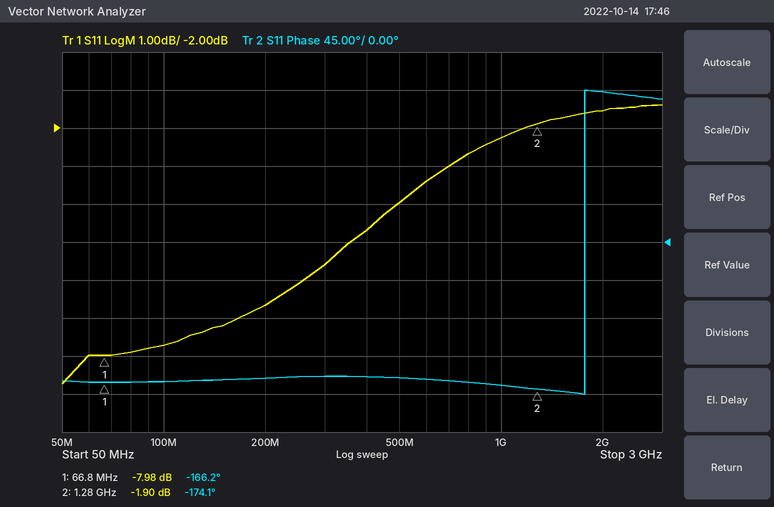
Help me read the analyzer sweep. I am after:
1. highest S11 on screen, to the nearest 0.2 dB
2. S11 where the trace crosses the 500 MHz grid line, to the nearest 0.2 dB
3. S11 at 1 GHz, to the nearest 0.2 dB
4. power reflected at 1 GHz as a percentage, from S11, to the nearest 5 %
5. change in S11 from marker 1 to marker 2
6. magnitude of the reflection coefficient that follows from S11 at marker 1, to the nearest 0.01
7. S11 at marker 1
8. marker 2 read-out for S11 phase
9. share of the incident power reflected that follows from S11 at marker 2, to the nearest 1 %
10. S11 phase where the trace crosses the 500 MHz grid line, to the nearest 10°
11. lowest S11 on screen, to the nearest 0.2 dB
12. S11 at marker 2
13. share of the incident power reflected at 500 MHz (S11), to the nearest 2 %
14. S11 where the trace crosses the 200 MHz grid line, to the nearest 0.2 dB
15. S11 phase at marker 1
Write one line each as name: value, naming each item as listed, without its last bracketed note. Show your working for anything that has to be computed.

highest S11 on screen, to the nearest 0.2 dB: -1.4 dB
S11 where the trace crosses the 500 MHz grid line, to the nearest 0.2 dB: -4.0 dB
S11 at 1 GHz, to the nearest 0.2 dB: -2.2 dB
power reflected at 1 GHz as a percentage, from S11, to the nearest 5 %: 10^(-2.2/10) ≈ 60 %
change in S11 from marker 1 to marker 2: -1.9 − (-7.98) = 6.08 dB
magnitude of the reflection coefficient that follows from S11 at marker 1, to the nearest 0.01: 10^(-7.98/20) ≈ 0.40
S11 at marker 1: -7.98 dB
marker 2 read-out for S11 phase: -174.1°
share of the incident power reflected that follows from S11 at marker 2, to the nearest 1 %: 10^(-1.9/10) ≈ 65 %
S11 phase where the trace crosses the 500 MHz grid line, to the nearest 10°: -160°
lowest S11 on screen, to the nearest 0.2 dB: -8.8 dB
S11 at marker 2: -1.90 dB
share of the incident power reflected at 500 MHz (S11), to the nearest 2 %: 10^(-4/10) ≈ 40 %
S11 where the trace crosses the 200 MHz grid line, to the nearest 0.2 dB: -6.6 dB
S11 phase at marker 1: -166.2°
